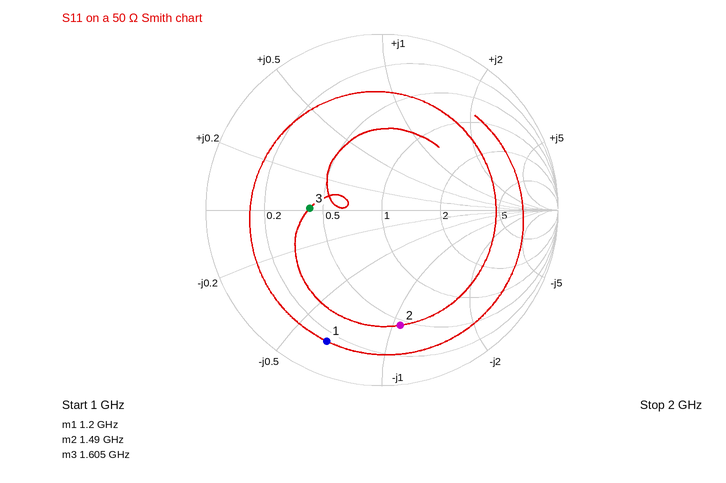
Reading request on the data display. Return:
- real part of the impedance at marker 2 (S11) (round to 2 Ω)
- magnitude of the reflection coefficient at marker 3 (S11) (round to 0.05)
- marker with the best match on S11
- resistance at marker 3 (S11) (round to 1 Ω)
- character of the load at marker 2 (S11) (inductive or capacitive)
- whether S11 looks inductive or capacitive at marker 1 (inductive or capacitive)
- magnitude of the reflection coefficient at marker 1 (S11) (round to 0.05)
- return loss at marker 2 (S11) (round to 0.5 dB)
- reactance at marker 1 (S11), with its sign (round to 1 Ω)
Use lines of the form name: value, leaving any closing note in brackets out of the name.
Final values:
real part of the impedance at marker 2 (S11): 22 Ω
magnitude of the reflection coefficient at marker 3 (S11): 0.40
marker with the best match on S11: marker 3
resistance at marker 3 (S11): 21 Ω
character of the load at marker 2 (S11): capacitive
whether S11 looks inductive or capacitive at marker 1: capacitive
magnitude of the reflection coefficient at marker 1 (S11): 0.80
return loss at marker 2 (S11): 3.5 dB
reactance at marker 1 (S11), with its sign: -33 Ω
